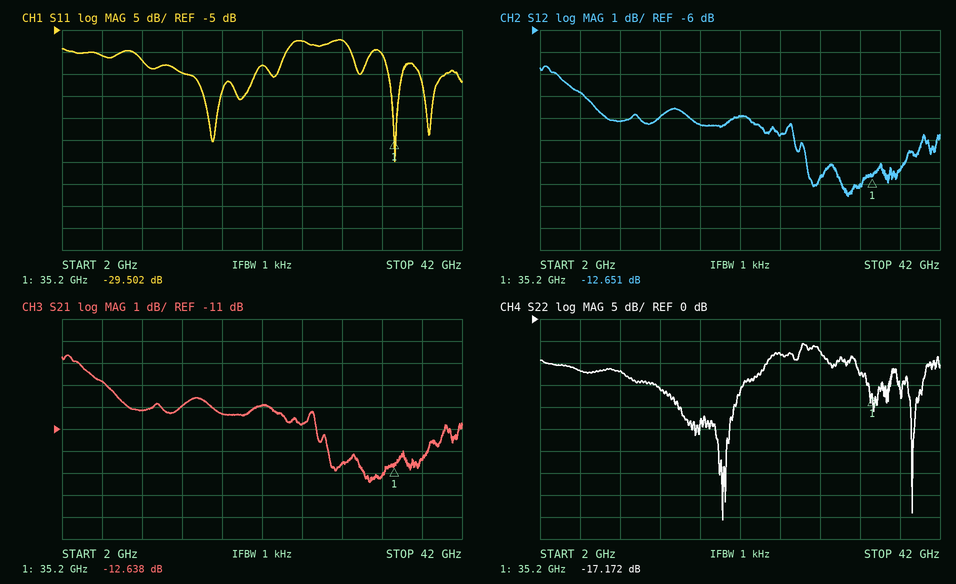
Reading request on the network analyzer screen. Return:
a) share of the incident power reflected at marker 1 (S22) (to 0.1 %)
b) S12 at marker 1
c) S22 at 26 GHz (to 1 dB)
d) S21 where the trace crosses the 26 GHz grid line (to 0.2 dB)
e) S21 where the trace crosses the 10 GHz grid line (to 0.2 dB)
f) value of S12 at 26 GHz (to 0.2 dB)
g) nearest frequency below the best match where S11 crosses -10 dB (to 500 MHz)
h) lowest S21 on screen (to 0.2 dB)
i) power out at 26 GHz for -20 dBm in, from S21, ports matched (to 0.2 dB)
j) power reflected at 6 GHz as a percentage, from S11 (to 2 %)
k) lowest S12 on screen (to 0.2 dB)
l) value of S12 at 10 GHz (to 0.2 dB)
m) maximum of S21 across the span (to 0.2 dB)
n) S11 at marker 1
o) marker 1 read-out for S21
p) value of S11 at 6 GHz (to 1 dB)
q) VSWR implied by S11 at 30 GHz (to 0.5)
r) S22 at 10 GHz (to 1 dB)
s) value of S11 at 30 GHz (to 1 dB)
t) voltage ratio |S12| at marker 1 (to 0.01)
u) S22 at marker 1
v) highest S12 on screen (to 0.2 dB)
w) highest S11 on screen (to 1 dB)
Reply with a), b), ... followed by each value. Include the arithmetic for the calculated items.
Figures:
a) 10^(-17.172/10) ≈ 1.9 %
b) -12.651 dB
c) -8 dB
d) -10.8 dB
e) -10.2 dB
f) -10.8 dB
g) 34.0 GHz
h) -13.4 dB
i) -20 dBm + (-10.8 dB) = -30.8 dBm
j) 10^(-11/10) ≈ 8 %
k) -13.6 dB
l) -10.2 dB
m) -7.6 dB
n) -29.502 dB
o) -12.638 dB
p) -11 dB
q) |Γ| = 10^(-7/20) = 0.4467; VSWR = (1 + 0.4467)/(1 − 0.4467) ≈ 2.61, so 2.5 to the nearest 0.5
r) -12 dB
s) -7 dB
t) 10^(-12.651/20) ≈ 0.23
u) -17.172 dB
v) -7.6 dB
w) -7 dB
